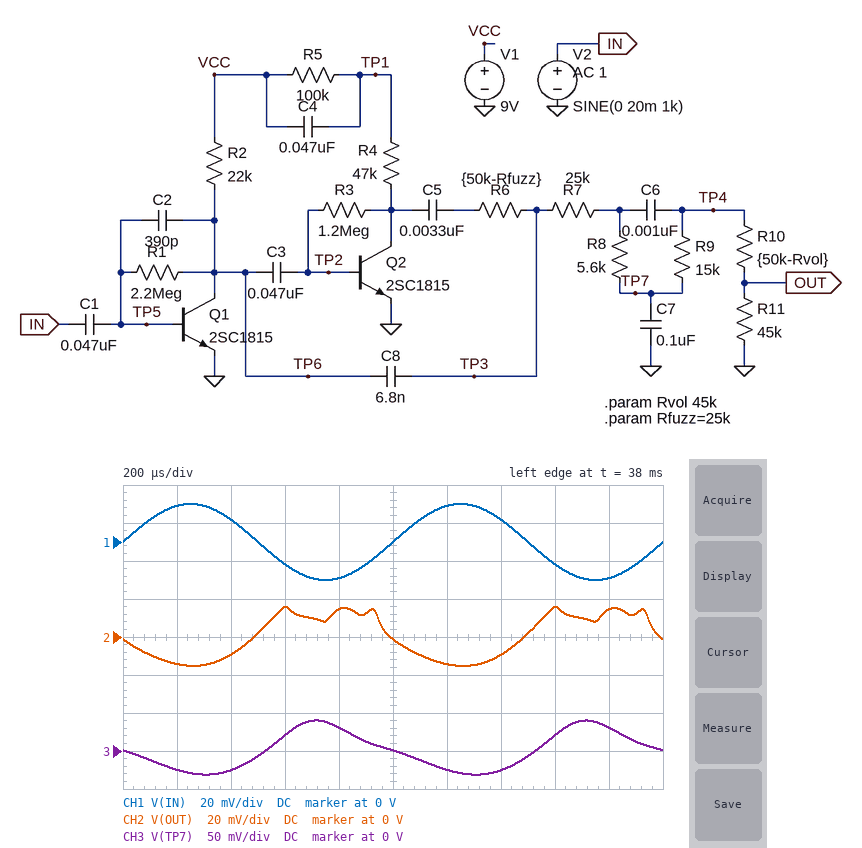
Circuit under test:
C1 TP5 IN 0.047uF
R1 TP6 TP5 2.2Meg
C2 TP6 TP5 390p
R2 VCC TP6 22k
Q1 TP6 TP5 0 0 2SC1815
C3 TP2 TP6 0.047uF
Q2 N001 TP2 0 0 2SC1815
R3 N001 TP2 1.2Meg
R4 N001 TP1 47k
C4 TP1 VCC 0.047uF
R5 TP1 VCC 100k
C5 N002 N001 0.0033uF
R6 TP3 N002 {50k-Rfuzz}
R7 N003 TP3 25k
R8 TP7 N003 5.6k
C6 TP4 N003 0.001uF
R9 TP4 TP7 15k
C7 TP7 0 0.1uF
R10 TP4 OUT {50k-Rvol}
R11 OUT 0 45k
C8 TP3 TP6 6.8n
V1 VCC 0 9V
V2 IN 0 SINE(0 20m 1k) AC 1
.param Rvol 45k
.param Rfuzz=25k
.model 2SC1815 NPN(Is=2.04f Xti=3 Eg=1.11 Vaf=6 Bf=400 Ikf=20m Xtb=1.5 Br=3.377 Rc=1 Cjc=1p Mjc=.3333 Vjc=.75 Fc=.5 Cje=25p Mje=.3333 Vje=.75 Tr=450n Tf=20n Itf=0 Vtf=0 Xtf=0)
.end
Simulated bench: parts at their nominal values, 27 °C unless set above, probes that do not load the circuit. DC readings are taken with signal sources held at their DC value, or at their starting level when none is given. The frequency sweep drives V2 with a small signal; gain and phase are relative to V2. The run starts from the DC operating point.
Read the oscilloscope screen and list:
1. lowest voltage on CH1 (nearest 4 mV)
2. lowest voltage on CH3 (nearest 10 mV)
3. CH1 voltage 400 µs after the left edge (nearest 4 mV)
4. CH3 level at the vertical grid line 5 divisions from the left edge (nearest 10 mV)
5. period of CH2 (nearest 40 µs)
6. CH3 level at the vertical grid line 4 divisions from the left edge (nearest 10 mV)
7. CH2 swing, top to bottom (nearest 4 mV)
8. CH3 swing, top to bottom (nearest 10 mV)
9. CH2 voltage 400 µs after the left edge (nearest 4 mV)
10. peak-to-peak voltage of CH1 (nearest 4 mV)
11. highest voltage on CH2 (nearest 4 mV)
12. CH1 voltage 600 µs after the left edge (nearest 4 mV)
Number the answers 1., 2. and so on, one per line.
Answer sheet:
1. -20 mV
2. -30 mV
3. 12 mV
4. 0 V
5. 1.00 ms
6. 30 mV
7. 32 mV
8. 70 mV
9. -8 mV
10. 40 mV
11. 16 mV
12. -12 mV
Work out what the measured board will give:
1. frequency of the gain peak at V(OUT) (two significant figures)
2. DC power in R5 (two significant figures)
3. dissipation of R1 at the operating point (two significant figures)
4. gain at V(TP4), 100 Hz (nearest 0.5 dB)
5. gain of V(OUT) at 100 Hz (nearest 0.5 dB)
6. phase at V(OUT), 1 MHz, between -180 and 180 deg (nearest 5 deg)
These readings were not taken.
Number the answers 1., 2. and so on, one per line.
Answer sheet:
1. 310 Hz
2. 310 µW
3. 910 nW
4. 29.0 dB
5. 28.0 dB
6. 105 deg
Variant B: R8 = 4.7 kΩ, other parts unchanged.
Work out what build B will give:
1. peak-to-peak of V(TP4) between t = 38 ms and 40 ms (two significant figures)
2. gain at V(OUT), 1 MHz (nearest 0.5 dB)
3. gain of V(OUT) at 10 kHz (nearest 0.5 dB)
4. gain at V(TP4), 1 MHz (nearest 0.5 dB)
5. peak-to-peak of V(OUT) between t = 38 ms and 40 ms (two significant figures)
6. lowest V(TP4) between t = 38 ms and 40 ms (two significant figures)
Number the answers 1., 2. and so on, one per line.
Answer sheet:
1. 36 mV
2. -8.5 dB
3. 4.5 dB
4. -7.5 dB
5. 33 mV
6. -18 mV
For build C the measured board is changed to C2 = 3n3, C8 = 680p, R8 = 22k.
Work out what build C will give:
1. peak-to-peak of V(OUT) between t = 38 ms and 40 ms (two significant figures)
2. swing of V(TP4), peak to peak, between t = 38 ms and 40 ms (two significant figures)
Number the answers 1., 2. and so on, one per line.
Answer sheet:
1. 200 mV
2. 220 mV
